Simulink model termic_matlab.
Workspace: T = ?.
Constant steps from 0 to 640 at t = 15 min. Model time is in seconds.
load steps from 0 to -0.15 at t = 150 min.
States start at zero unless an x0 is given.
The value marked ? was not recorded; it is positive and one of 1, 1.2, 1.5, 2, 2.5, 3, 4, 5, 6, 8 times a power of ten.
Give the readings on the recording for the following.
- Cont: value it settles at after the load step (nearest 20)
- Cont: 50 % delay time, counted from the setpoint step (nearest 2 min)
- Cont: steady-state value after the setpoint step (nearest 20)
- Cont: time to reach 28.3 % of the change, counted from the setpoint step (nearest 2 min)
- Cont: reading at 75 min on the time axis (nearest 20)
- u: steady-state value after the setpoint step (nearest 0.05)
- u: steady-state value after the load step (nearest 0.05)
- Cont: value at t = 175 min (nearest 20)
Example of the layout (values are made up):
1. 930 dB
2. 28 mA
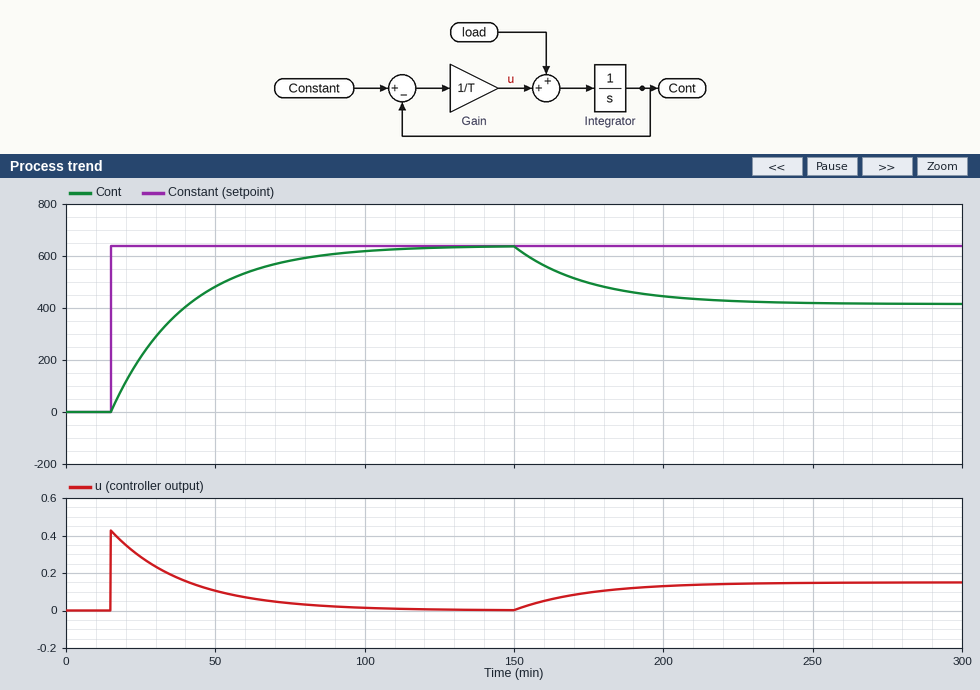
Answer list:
1. 420
2. 18 min
3. 640
4. 8 min
5. 580
6. 0.00
7. 0.15
8. 500
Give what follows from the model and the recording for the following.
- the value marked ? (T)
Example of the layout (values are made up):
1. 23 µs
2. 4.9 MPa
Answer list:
1. 1500
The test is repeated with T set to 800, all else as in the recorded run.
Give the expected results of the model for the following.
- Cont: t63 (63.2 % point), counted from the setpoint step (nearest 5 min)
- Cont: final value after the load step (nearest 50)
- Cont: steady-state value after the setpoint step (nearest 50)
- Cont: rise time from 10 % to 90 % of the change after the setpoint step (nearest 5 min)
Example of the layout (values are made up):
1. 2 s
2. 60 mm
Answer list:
1. 15 min
2. 500
3. 650
4. 30 min
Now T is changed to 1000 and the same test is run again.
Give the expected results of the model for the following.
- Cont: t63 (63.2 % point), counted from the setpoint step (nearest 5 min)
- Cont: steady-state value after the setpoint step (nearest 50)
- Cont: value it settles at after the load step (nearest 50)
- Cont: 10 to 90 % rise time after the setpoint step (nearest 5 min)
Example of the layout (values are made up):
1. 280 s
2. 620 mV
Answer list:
1. 15 min
2. 650
3. 500
4. 35 min
